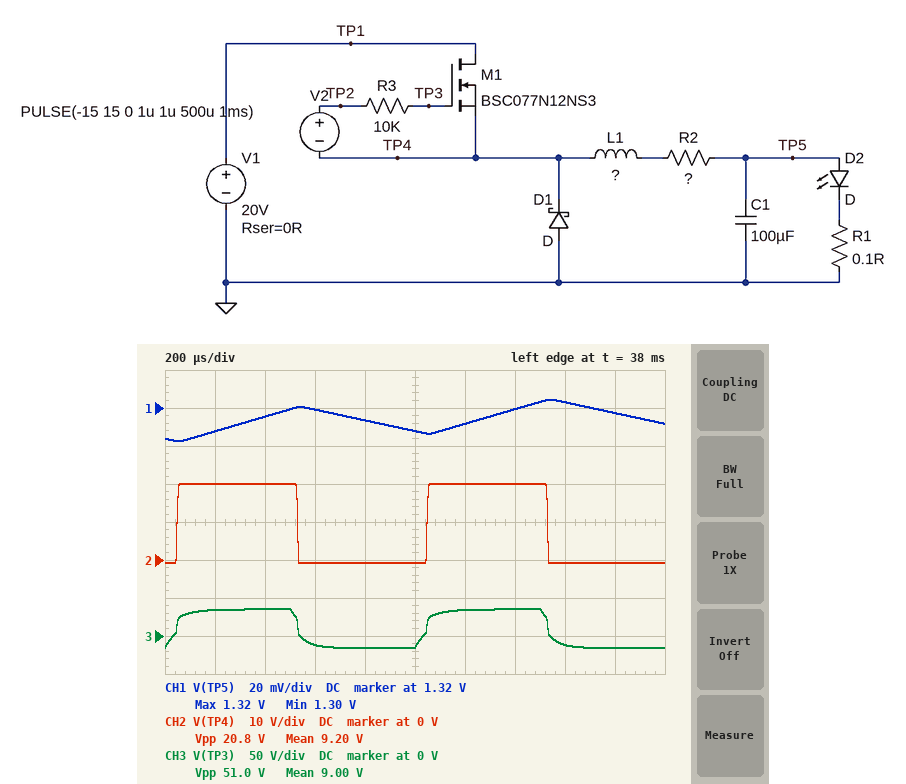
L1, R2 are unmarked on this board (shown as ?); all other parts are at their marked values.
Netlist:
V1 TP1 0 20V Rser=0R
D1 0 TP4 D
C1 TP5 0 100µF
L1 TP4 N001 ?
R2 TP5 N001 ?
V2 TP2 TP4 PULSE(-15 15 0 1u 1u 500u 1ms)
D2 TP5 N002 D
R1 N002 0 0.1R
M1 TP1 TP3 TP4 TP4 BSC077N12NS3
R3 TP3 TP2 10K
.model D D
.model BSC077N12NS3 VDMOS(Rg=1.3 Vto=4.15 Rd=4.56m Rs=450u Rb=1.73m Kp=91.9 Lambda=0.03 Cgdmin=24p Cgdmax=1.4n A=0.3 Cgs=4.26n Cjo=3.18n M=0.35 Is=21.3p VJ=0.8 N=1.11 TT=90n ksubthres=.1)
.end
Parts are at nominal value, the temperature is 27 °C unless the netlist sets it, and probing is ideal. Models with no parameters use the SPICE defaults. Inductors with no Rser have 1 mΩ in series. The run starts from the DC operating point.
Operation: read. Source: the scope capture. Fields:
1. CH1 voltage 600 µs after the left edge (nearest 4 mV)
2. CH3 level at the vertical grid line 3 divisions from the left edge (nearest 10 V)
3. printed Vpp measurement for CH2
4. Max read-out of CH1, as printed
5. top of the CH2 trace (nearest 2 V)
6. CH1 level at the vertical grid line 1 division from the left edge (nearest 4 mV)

1.320 V
-10 V
20.8 V
1.32 V
20 V
1.308 V
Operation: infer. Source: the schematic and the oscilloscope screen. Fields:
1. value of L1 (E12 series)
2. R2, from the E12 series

33 mH
1.5 Ω
